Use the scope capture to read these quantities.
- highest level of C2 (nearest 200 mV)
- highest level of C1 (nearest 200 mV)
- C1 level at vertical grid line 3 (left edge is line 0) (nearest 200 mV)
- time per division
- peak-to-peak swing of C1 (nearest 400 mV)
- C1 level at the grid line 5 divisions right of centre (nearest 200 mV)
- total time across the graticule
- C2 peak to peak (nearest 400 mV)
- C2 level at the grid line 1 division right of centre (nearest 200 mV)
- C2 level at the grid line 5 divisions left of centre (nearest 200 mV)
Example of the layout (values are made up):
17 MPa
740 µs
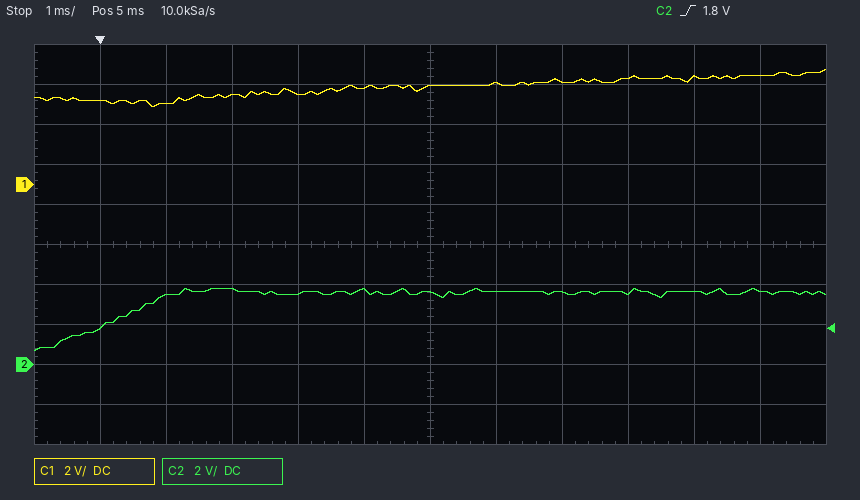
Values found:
3.8 V
5.8 V
4.4 V
1 ms
2.0 V
5.4 V
12 ms
3.2 V
3.6 V
1.8 V
